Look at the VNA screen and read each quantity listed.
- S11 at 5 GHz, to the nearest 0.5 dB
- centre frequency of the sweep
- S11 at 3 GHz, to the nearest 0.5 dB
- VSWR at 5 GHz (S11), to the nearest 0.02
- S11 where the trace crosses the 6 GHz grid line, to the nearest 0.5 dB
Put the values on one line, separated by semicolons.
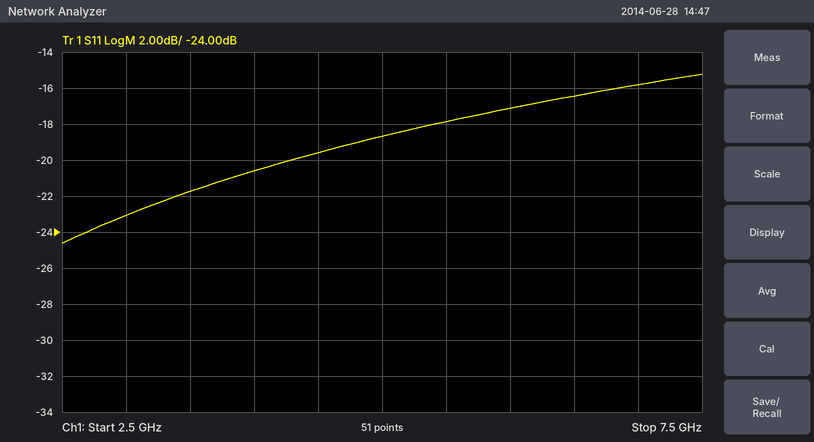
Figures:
-18.5 dB; 5 GHz; -23.0 dB; 1.26; -17.0 dB
